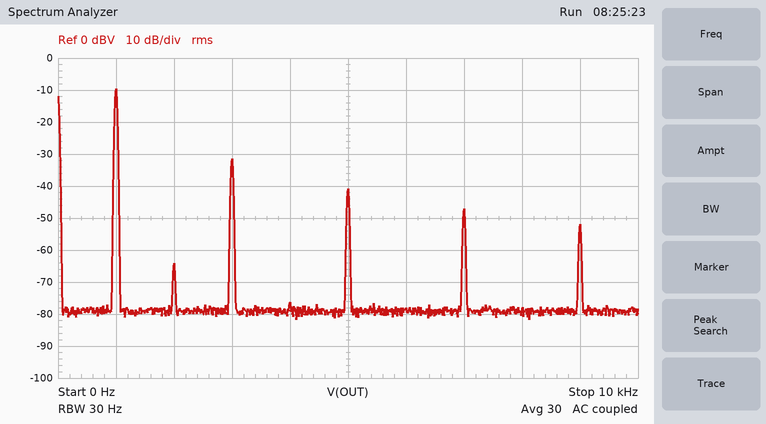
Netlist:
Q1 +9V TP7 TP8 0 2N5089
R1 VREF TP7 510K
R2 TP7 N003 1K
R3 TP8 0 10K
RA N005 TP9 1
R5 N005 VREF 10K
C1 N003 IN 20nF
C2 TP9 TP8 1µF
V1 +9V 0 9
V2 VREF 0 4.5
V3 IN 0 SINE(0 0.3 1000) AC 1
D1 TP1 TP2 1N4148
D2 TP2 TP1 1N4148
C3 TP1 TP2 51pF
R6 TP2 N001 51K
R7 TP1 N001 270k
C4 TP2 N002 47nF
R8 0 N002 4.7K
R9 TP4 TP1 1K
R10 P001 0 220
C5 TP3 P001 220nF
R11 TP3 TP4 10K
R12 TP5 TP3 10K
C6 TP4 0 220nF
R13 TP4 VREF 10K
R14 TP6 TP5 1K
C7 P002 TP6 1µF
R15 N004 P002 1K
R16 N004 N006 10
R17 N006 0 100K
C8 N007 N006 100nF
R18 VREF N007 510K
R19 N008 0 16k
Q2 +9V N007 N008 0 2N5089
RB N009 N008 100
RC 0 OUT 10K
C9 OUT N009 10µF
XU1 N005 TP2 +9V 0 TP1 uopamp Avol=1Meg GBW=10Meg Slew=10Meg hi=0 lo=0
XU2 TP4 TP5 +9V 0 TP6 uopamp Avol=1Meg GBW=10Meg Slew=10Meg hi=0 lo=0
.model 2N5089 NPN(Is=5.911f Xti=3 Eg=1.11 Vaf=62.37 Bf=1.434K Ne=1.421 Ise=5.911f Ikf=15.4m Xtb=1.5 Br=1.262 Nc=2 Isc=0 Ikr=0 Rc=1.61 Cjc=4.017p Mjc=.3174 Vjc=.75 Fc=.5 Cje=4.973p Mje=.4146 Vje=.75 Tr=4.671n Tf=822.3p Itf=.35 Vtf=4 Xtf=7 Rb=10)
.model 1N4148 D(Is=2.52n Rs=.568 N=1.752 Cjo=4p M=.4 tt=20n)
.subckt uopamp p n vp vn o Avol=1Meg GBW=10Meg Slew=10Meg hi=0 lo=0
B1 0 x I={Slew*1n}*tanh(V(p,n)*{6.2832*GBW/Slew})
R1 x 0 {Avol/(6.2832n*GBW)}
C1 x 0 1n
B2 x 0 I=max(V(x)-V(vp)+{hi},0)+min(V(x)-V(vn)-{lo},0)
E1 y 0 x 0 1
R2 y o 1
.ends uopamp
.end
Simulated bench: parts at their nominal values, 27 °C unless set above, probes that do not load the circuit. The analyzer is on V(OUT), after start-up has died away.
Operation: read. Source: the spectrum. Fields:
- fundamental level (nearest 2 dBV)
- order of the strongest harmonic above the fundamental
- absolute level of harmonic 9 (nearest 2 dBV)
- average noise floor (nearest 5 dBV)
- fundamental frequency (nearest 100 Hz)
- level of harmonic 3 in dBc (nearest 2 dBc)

-10 dBV
3
-52 dBV
-80 dBV
1.0 kHz
-22 dBc
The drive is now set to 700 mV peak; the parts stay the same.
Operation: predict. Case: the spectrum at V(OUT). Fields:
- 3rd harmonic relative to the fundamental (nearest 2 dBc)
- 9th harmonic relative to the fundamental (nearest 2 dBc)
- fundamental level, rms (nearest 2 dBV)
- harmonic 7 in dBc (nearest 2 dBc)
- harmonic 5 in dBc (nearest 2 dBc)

-24 dBc
-44 dBc
-6 dBV
-40 dBc
-34 dBc
